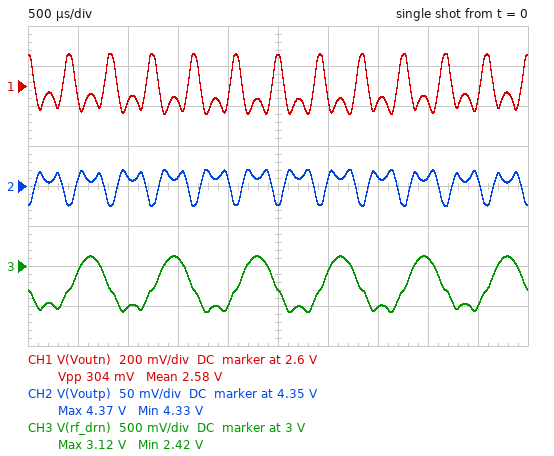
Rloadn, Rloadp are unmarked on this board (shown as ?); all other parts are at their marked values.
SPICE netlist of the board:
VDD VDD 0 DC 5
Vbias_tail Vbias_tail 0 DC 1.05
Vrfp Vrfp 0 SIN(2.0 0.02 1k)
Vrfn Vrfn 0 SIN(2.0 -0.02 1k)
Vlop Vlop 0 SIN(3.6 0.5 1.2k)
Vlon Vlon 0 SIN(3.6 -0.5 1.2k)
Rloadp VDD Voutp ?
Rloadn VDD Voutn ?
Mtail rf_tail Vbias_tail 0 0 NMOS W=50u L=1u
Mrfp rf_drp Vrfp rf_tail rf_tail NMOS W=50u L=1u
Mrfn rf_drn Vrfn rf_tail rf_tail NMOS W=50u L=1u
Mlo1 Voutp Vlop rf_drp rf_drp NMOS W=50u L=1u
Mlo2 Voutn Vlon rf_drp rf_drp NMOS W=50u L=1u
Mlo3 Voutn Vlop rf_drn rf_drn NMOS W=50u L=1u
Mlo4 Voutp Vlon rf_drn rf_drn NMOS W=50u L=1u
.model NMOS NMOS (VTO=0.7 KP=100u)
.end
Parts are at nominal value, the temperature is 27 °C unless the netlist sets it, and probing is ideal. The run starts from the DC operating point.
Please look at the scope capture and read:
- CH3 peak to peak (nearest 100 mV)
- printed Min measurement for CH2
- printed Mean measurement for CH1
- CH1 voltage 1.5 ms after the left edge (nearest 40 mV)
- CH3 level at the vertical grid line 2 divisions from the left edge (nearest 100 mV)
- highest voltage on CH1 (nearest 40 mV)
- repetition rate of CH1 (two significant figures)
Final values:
700 mV
4.33 V
2.58 V
2.52 V
2.5 V
2.76 V
2.4 kHz
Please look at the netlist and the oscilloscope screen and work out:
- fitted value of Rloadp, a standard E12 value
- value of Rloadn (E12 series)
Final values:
3.3 kΩ
22 kΩ
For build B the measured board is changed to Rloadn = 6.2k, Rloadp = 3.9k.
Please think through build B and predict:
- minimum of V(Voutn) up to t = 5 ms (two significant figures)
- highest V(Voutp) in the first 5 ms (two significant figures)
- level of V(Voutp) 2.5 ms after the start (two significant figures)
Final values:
3.9 V
4.5 V
4.4 V
